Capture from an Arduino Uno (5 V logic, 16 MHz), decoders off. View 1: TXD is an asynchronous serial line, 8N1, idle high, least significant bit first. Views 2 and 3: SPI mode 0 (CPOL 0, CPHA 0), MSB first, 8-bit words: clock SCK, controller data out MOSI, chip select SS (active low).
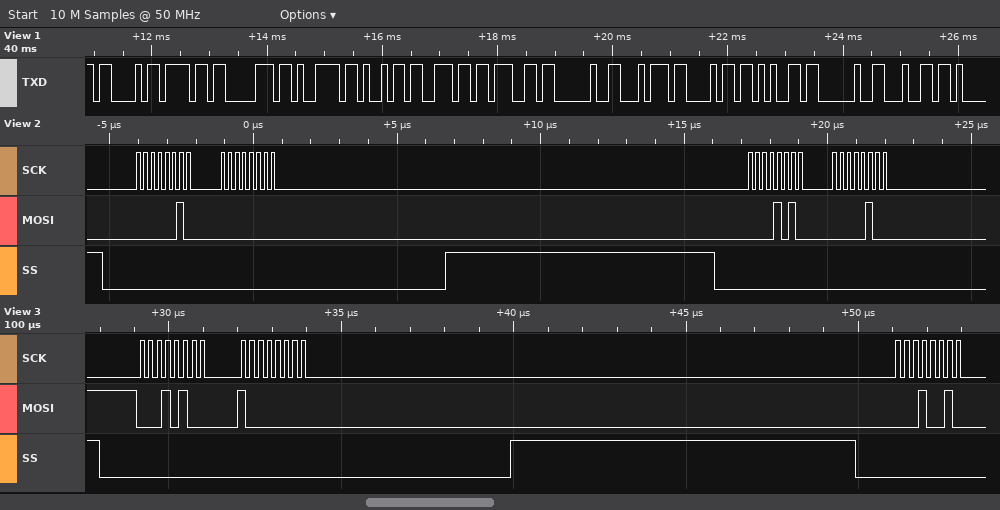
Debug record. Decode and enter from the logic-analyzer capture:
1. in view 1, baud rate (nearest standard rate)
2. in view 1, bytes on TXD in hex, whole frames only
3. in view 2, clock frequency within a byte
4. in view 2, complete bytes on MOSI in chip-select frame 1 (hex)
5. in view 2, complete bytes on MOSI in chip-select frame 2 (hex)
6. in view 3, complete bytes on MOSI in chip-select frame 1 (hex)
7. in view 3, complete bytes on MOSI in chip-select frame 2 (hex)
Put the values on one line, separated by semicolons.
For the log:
9600 baud; 0x43 0x6F 0x70 0x79 0x69 0x6E 0x67 0x20 0x74 0x68 0x65 0x20 0x64; 4 MHz; 0x02 0x00; 0x0A 0x04; 14 80; 12
